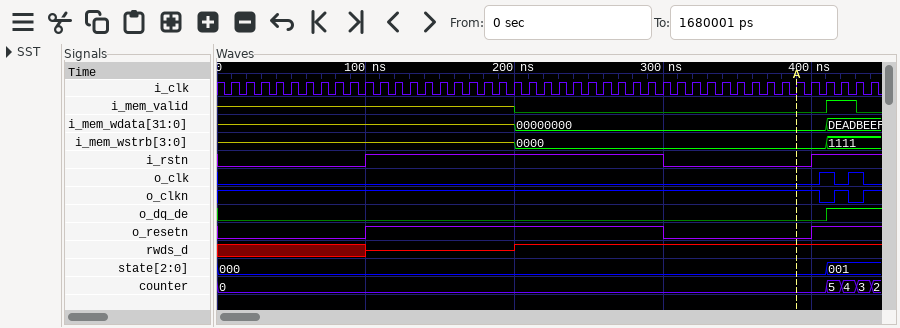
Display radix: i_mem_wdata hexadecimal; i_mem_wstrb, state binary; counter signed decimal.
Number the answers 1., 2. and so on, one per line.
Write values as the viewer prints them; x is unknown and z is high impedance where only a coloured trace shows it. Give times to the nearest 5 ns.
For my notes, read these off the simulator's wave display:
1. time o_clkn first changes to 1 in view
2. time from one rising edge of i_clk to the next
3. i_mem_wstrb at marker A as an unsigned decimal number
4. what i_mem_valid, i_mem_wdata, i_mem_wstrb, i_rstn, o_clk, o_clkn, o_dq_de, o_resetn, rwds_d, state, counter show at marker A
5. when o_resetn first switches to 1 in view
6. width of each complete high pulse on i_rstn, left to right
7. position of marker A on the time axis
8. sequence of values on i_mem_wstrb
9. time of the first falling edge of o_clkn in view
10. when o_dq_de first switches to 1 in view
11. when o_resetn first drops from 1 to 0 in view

1. 415 ns
2. 10 ns
3. 0
4. i_mem_valid=0, i_mem_wdata=00000000, i_mem_wstrb=0000, i_rstn=0, o_clk=0, o_clkn=1, o_dq_de=0, o_resetn=0, rwds_d=1, state=000, counter=0
5. 100 ns
6. 200 ns
7. 390 ns
8. z, 0000, 1111
9. 405 ns
10. 410 ns
11. 300 ns
